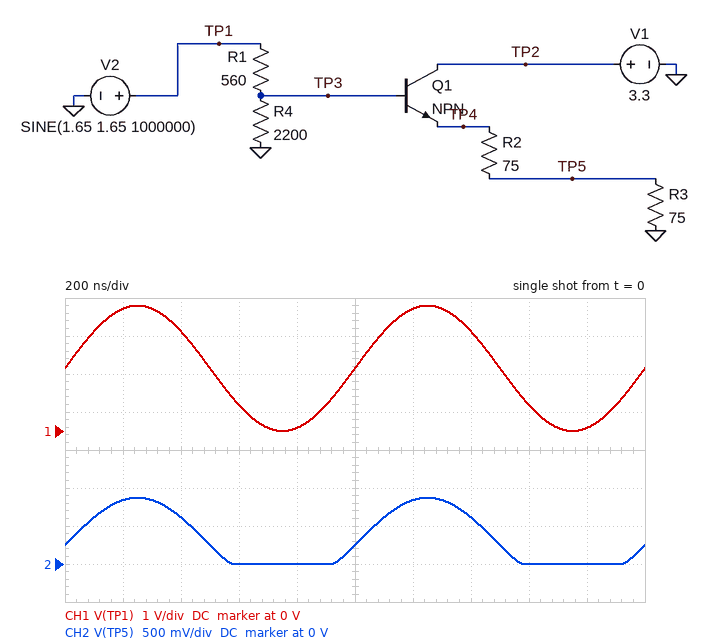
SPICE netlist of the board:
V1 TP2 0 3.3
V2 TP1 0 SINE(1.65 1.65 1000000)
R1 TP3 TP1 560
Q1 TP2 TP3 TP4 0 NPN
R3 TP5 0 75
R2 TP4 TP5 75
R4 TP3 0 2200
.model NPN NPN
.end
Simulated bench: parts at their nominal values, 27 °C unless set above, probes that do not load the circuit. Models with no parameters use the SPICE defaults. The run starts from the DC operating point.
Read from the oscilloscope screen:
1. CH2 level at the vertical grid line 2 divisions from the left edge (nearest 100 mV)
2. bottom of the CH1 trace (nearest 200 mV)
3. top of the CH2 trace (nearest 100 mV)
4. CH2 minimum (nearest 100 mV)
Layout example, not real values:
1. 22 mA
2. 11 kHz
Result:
1. 600 mV
2. 0 V
3. 900 mV
4. 0 V
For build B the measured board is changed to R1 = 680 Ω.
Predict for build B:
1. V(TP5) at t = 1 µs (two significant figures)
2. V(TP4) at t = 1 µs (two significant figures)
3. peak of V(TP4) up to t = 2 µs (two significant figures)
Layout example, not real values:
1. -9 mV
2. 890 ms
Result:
1. 220 mV
2. 440 mV
3. 1.6 V
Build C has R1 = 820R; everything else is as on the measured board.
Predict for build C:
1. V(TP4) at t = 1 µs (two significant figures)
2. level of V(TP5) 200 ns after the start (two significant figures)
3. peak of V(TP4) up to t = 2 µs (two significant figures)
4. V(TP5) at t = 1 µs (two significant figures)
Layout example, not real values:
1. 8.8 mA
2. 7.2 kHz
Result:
1. 390 mV
2. 730 mV
3. 1.5 V
4. 190 mV
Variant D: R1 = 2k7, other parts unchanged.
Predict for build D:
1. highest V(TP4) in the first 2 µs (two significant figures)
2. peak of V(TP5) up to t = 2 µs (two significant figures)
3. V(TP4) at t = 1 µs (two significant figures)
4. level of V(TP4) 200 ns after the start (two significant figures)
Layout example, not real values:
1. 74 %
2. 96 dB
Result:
1. 620 mV
2. 310 mV
3. 19 mV
4. 590 mV
